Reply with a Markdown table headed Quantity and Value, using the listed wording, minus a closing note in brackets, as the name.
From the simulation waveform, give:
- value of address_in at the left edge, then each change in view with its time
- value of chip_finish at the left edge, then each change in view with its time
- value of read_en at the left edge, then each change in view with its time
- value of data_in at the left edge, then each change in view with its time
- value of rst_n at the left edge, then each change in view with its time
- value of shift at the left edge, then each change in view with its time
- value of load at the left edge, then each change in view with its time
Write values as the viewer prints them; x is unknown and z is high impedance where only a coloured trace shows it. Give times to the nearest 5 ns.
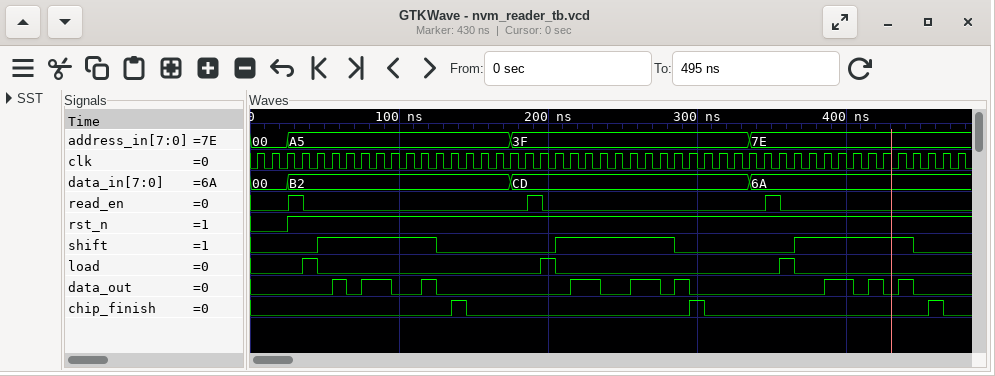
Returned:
| Quantity | Value |
|---|---|
| value of address_in at the left edge, then each change in view with its time | 00, A5 at 25 ns, 3F at 175 ns, 7E at 335 ns |
| value of chip_finish at the left edge, then each change in view with its time | 0, 1 at 135 ns, 0 at 145 ns, 1 at 295 ns, 0 at 305 ns, 1 at 455 ns, 0 at 465 ns |
| value of read_en at the left edge, then each change in view with its time | 0, 1 at 25 ns, 0 at 35 ns, 1 at 185 ns, 0 at 195 ns, 1 at 345 ns, 0 at 355 ns |
| value of data_in at the left edge, then each change in view with its time | 00, B2 at 25 ns, CD at 175 ns, 6A at 335 ns |
| value of rst_n at the left edge, then each change in view with its time | 0, 1 at 25 ns |
| value of shift at the left edge, then each change in view with its time | 0, 1 at 45 ns, 0 at 125 ns, 1 at 205 ns, 0 at 285 ns, 1 at 365 ns, 0 at 445 ns |
| value of load at the left edge, then each change in view with its time | 0, 1 at 35 ns, 0 at 45 ns, 1 at 195 ns, 0 at 205 ns, 1 at 355 ns, 0 at 365 ns |
